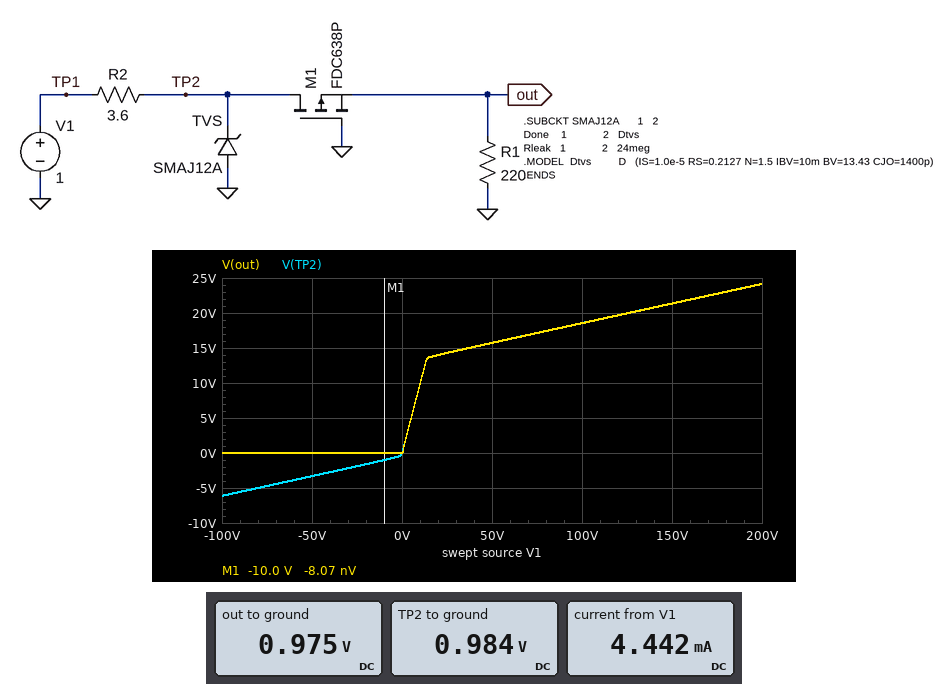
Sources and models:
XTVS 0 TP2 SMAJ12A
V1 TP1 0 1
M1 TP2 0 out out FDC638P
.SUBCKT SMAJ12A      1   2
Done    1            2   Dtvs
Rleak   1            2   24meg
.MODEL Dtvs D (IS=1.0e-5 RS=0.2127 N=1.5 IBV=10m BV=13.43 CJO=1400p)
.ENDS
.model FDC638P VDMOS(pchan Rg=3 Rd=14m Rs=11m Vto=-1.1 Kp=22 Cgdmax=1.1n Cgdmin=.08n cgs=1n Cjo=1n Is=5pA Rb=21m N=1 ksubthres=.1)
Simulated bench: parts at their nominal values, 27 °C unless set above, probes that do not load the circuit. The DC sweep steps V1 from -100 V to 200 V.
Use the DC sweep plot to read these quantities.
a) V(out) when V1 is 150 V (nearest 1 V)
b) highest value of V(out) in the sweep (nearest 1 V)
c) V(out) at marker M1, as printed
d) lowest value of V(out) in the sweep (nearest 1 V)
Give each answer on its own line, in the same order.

21 V
24 V
-8.07 nV
0 V
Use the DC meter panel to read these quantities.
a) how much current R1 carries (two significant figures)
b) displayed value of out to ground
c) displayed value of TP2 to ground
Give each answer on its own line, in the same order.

4.4 mA
0.975 V
0.984 V
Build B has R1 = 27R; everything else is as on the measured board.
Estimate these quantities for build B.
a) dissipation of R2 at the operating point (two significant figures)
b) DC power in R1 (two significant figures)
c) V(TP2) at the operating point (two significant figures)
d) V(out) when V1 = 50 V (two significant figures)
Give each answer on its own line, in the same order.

760 µW
5.7 mW
950 mV
16 V
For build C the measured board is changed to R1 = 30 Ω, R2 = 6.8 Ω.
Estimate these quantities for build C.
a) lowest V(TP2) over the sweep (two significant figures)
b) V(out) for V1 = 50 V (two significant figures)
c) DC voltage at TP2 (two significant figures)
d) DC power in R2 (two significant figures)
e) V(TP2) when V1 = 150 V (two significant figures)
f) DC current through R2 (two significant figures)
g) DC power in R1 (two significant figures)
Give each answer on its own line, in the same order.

-3.6 V
15 V
920 mV
1.0 mW
18 V
12 mA
4.4 mW
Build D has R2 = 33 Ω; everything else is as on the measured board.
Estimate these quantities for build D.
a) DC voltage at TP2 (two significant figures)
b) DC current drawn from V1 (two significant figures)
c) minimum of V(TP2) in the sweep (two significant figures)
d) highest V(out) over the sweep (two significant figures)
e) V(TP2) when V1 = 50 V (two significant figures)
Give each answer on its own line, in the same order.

920 mV
2.5 mA
-1.1 V
15 V
14 V
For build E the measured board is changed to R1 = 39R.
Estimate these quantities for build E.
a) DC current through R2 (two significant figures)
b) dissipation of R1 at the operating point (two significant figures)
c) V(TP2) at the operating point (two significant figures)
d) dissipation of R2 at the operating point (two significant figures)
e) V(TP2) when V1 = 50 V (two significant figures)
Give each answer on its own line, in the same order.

11 mA
4.6 mW
960 mV
420 µW
16 V
